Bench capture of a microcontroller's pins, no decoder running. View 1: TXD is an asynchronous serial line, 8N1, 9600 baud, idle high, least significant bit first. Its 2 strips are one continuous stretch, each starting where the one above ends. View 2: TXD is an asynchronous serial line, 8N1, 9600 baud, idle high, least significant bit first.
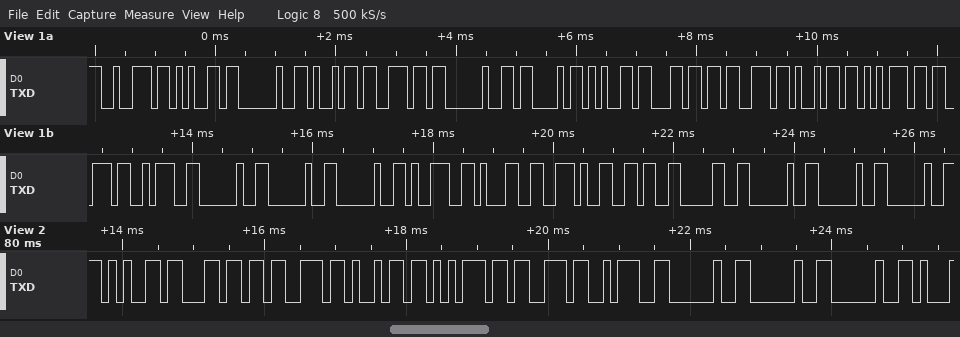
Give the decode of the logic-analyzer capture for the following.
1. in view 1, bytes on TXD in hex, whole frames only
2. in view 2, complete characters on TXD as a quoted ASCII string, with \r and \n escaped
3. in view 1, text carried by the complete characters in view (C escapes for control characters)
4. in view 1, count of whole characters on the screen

72 65 20 69 6E 20 43 65 6C 73 69 75 73 3A 20 20 20 39 31 2E 36 30 20 20 20
"elsius:   "
"re in Celsius:   91.60   "
25
